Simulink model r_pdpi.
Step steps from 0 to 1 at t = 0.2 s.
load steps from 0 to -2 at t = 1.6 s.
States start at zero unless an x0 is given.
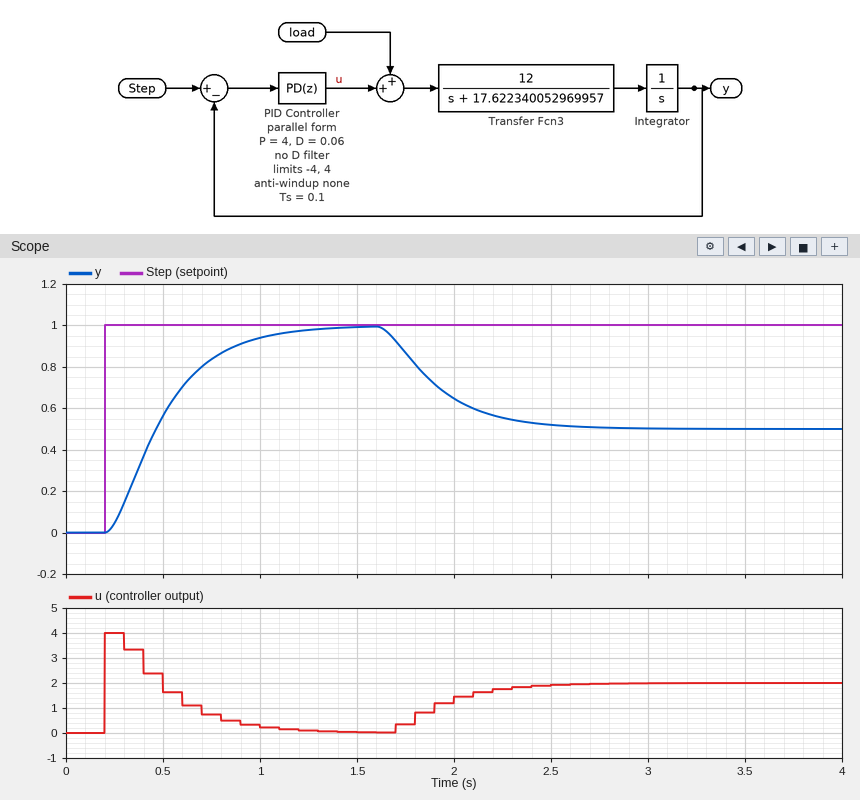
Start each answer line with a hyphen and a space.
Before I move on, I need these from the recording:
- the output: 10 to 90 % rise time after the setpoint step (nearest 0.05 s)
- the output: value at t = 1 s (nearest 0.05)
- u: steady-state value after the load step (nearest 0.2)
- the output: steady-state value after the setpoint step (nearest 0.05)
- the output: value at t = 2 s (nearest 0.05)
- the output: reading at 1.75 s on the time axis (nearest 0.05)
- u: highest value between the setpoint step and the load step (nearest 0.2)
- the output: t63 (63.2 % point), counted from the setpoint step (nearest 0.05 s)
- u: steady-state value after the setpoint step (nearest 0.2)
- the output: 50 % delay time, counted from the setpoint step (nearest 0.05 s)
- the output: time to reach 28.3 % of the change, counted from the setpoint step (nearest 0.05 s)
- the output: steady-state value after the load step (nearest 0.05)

- 0.60 s
- 0.95
- 2.0
- 1.00
- 0.65
- 0.85
- 4.0
- 0.35 s
- 0.0
- 0.25 s
- 0.15 s
- 0.50
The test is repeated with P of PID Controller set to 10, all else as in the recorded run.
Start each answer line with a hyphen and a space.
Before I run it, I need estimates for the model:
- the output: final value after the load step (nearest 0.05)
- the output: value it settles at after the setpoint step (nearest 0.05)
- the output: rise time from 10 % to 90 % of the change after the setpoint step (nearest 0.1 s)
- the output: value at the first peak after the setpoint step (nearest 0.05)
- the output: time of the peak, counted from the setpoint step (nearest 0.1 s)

- 0.80
- 1.00
- 0.3 s
- 1.05
- 0.6 s
